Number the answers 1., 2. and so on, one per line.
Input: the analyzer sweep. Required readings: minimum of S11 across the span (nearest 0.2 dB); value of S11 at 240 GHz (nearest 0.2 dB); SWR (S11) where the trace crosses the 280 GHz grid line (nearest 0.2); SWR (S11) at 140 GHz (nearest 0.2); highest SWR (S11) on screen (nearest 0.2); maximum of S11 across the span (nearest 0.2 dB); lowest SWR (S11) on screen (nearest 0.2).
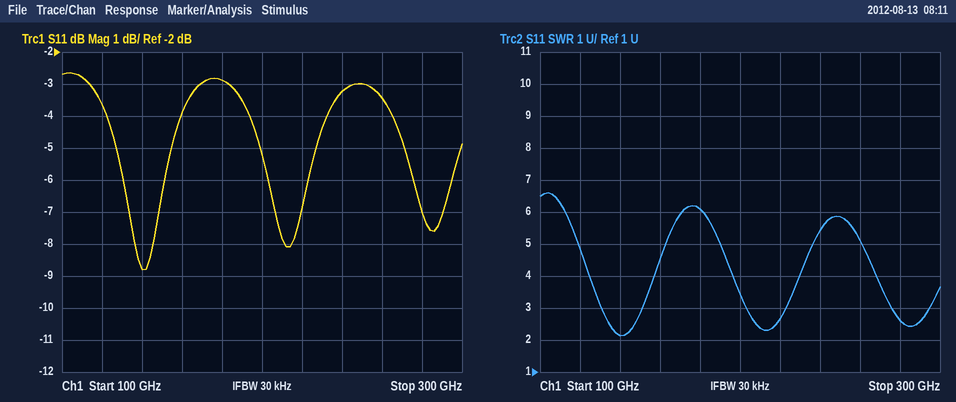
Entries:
1. -8.8 dB
2. -3.2 dB
3. 2.6
4. 2.2
5. 6.6
6. -2.6 dB
7. 2.2
